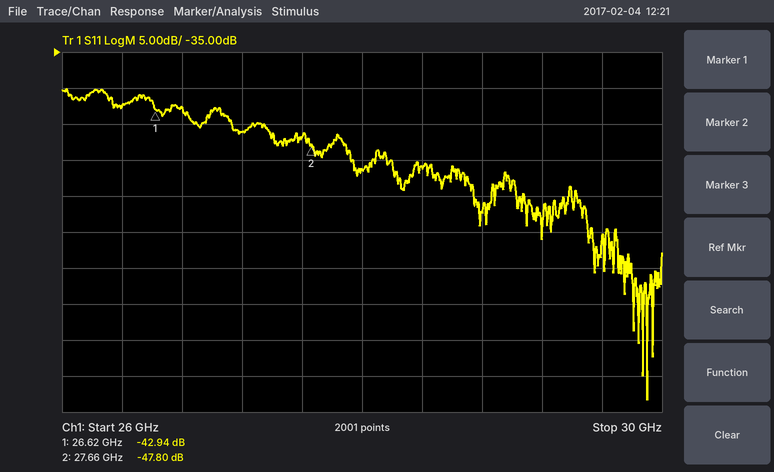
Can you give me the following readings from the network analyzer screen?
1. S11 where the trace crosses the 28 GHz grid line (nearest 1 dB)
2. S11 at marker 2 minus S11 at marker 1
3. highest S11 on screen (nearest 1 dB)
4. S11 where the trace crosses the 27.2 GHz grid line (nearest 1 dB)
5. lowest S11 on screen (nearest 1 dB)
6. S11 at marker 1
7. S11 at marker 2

-51 dB
-4.86 dB
-40 dB
-46 dB
-83 dB
-42.94 dB
-47.80 dB
